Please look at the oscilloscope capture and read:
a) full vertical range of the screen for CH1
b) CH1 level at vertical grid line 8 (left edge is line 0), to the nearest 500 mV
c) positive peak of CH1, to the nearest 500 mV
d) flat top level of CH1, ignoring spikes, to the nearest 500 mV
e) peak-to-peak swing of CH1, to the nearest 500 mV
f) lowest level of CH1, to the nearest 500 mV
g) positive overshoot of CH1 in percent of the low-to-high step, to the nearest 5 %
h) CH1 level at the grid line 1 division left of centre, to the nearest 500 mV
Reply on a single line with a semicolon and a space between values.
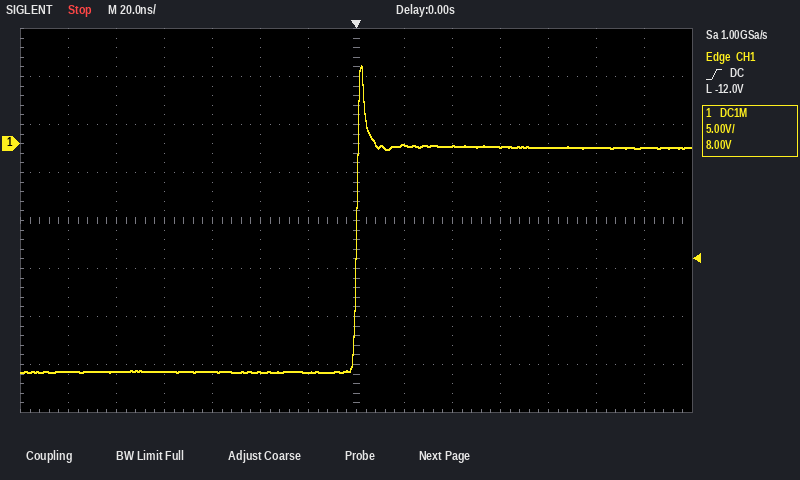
40 V; 0.0 V; 8.0 V; -500 mV; 32.0 V; -24.0 V; 35 %; -24.0 V
